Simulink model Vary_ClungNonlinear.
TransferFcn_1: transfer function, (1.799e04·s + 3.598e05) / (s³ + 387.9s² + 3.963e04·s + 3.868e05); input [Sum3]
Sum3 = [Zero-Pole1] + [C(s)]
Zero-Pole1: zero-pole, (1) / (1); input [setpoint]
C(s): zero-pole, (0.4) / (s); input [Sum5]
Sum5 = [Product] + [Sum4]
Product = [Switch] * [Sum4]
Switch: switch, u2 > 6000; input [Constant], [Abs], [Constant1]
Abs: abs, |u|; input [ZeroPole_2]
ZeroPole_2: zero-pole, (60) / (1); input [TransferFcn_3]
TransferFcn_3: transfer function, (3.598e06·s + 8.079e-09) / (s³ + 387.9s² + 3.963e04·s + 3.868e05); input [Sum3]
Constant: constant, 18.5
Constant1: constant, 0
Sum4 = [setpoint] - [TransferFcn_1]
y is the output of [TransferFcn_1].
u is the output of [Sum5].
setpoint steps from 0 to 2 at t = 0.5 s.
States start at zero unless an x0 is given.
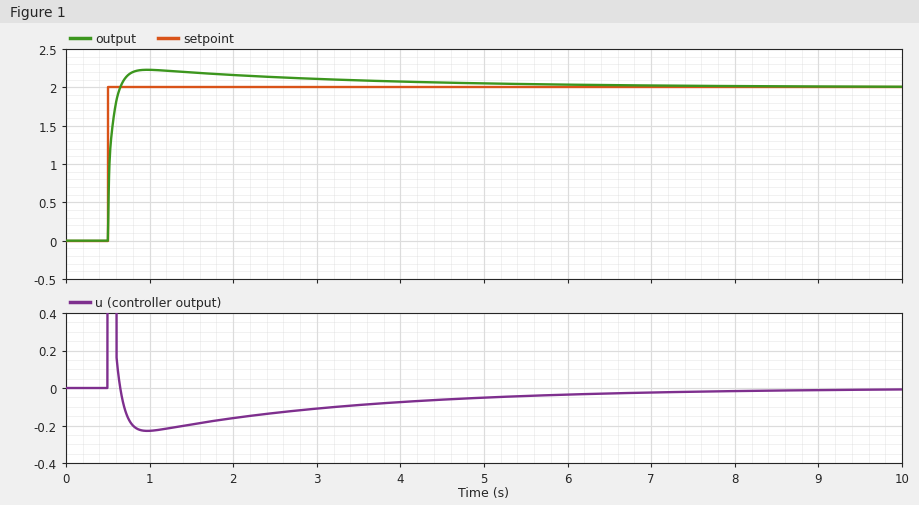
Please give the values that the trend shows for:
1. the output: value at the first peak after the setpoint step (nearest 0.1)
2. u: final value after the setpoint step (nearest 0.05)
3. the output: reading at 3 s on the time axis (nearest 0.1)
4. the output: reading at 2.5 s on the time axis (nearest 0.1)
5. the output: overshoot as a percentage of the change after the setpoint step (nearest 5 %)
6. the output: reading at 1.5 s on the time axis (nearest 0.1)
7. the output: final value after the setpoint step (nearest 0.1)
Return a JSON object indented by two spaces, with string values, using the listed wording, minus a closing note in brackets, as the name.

{
  "the output: value at the first peak after the setpoint step": "2.2",
  "u: final value after the setpoint step": "0.00",
  "the output: reading at 3 s on the time axis": "2.1",
  "the output: reading at 2.5 s on the time axis": "2.1",
  "the output: overshoot as a percentage of the change after the setpoint step": "10 %",
  "the output: reading at 1.5 s on the time axis": "2.2",
  "the output: final value after the setpoint step": "2.0"
}
